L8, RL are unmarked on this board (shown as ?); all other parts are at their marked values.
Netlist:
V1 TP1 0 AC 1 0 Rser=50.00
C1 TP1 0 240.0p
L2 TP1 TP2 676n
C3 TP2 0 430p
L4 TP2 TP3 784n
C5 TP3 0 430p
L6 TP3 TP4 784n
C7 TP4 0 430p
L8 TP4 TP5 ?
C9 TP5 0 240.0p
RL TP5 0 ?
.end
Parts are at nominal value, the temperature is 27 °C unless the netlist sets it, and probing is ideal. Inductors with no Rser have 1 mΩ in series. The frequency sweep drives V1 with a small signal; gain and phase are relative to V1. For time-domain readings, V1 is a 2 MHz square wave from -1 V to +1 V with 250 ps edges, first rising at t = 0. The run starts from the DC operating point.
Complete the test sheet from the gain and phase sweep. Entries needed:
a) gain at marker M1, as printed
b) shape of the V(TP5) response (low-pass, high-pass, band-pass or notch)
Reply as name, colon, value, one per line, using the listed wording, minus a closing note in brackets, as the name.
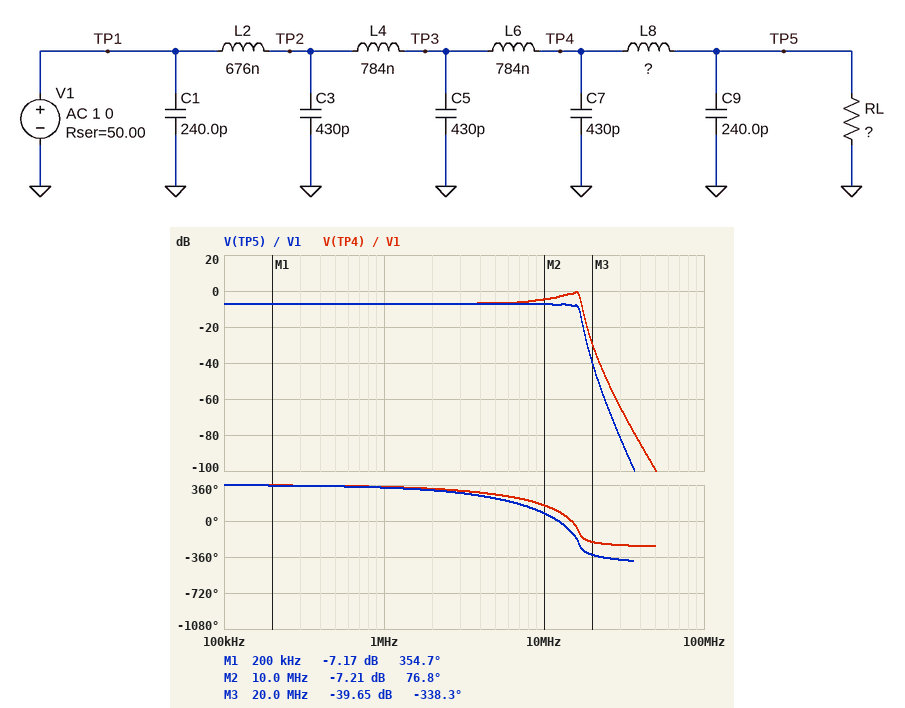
gain at marker M1, as printed: -7.17 dB
shape of the V(TP5) response: low-pass
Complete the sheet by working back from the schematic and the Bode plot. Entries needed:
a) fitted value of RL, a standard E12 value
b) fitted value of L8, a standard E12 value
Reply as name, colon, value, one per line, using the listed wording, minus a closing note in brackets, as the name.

fitted value of RL, a standard E12 value: 39 Ω
fitted value of L8, a standard E12 value: 820 nH
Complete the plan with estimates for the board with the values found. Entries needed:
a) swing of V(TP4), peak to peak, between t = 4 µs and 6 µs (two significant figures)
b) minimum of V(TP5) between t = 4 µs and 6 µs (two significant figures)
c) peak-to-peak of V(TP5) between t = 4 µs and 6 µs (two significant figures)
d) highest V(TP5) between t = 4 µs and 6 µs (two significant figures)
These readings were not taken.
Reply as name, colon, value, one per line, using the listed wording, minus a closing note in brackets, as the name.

swing of V(TP4), peak to peak, between t = 4 µs and 6 µs: 1.4 V
minimum of V(TP5) between t = 4 µs and 6 µs: -600 mV
peak-to-peak of V(TP5) between t = 4 µs and 6 µs: 1.2 V
highest V(TP5) between t = 4 µs and 6 µs: 600 mV
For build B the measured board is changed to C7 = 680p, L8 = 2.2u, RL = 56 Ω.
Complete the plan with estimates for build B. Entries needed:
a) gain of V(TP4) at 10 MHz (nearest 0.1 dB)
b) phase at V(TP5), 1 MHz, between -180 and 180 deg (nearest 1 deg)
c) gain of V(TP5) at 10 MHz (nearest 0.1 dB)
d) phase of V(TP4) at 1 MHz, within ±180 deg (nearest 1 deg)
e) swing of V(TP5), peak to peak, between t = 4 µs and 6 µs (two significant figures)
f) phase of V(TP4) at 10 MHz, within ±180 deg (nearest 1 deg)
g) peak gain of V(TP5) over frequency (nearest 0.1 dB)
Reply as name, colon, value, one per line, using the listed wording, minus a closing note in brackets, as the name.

gain of V(TP4) at 10 MHz: -4.5 dB
phase at V(TP5), 1 MHz, between -180 and 180 deg: -34 deg
gain of V(TP5) at 10 MHz: -13.1 dB
phase of V(TP4) at 1 MHz, within ±180 deg: -20 deg
swing of V(TP5), peak to peak, between t = 4 µs and 6 µs: 1.2 V
phase of V(TP4) at 10 MHz, within ±180 deg: 110 deg
peak gain of V(TP5) over frequency: -5.5 dB
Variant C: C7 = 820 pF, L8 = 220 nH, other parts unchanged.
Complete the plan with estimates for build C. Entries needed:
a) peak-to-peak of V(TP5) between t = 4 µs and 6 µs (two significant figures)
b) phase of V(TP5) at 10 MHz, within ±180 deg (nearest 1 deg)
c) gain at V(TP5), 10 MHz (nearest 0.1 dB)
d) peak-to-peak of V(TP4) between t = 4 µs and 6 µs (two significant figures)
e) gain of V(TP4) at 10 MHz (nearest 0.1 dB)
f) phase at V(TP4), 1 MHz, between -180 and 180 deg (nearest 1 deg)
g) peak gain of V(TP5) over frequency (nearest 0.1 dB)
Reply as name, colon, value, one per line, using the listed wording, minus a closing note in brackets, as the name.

peak-to-peak of V(TP5) between t = 4 µs and 6 µs: 990 mV
phase of V(TP5) at 10 MHz, within ±180 deg: 93 deg
gain at V(TP5), 10 MHz: -9.8 dB
peak-to-peak of V(TP4) between t = 4 µs and 6 µs: 920 mV
gain of V(TP4) at 10 MHz: -11.0 dB
phase at V(TP4), 1 MHz, between -180 and 180 deg: -25 deg
peak gain of V(TP5) over frequency: -7.2 dB
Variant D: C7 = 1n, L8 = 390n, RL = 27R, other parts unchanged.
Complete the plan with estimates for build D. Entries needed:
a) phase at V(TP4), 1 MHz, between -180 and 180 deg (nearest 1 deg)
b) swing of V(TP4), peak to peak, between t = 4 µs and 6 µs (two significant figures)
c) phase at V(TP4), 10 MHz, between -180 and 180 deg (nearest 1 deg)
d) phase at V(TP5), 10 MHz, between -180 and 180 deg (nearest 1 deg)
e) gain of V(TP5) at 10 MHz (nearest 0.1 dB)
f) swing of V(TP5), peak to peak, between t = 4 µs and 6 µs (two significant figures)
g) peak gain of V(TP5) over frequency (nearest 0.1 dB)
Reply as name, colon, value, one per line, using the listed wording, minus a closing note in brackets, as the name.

phase at V(TP4), 1 MHz, between -180 and 180 deg: -22 deg
swing of V(TP4), peak to peak, between t = 4 µs and 6 µs: 940 mV
phase at V(TP4), 10 MHz, between -180 and 180 deg: 124 deg
phase at V(TP5), 10 MHz, between -180 and 180 deg: 69 deg
gain of V(TP5) at 10 MHz: -10.5 dB
swing of V(TP5), peak to peak, between t = 4 µs and 6 µs: 910 mV
peak gain of V(TP5) over frequency: -8.9 dB
